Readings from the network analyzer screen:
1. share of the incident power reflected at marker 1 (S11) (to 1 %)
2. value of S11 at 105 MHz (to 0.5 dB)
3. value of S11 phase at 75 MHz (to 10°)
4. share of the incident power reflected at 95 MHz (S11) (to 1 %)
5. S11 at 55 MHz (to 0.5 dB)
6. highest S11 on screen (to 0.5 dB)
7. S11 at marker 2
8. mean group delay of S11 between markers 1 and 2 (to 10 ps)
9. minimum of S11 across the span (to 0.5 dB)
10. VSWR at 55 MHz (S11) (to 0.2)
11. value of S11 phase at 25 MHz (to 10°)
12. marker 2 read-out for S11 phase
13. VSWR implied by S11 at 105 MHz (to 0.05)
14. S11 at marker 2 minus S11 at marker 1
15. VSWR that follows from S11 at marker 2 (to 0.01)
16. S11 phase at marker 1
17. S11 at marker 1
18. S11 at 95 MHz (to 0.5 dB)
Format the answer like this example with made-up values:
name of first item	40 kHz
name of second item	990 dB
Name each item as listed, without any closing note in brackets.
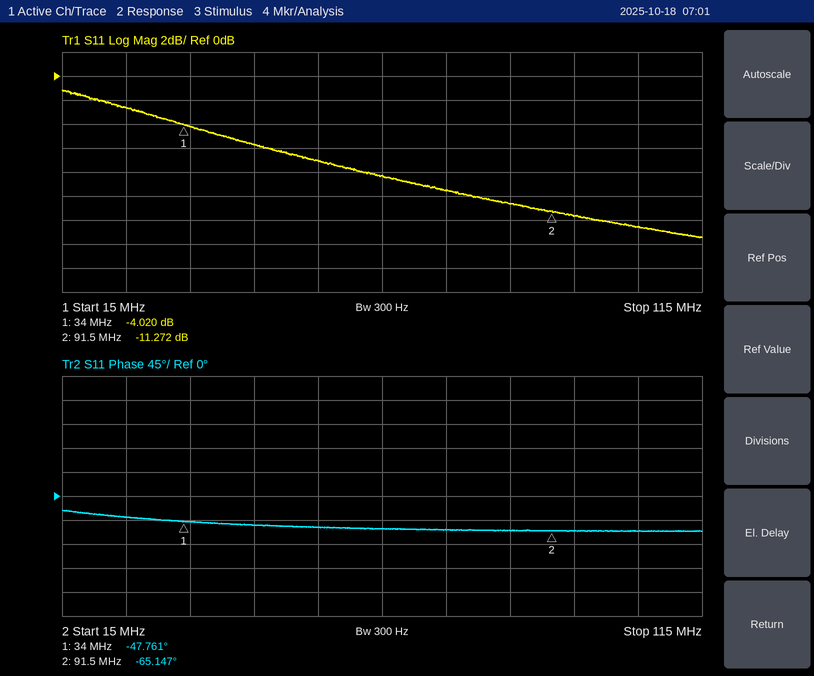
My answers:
share of the incident power reflected at marker 1 (S11)	40 %
value of S11 at 105 MHz	-12.5 dB
value of S11 phase at 75 MHz	-60°
share of the incident power reflected at 95 MHz (S11)	7 %
S11 at 55 MHz	-7.0 dB
highest S11 on screen	-1.0 dB
S11 at marker 2	-11.272 dB
mean group delay of S11 between markers 1 and 2	840 ps
minimum of S11 across the span	-13.5 dB
VSWR at 55 MHz (S11)	2.6
value of S11 phase at 25 MHz	-40°
marker 2 read-out for S11 phase	-65.147°
VSWR implied by S11 at 105 MHz	1.60
S11 at marker 2 minus S11 at marker 1	-7.252 dB
VSWR that follows from S11 at marker 2	1.75
S11 phase at marker 1	-47.761°
S11 at marker 1	-4.020 dB
S11 at 95 MHz	-11.5 dB
